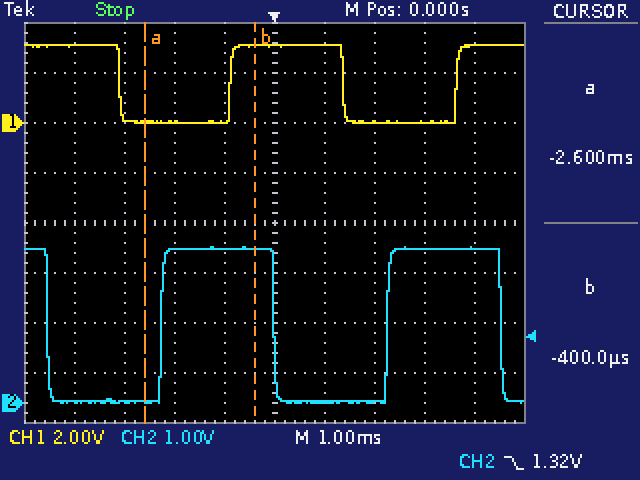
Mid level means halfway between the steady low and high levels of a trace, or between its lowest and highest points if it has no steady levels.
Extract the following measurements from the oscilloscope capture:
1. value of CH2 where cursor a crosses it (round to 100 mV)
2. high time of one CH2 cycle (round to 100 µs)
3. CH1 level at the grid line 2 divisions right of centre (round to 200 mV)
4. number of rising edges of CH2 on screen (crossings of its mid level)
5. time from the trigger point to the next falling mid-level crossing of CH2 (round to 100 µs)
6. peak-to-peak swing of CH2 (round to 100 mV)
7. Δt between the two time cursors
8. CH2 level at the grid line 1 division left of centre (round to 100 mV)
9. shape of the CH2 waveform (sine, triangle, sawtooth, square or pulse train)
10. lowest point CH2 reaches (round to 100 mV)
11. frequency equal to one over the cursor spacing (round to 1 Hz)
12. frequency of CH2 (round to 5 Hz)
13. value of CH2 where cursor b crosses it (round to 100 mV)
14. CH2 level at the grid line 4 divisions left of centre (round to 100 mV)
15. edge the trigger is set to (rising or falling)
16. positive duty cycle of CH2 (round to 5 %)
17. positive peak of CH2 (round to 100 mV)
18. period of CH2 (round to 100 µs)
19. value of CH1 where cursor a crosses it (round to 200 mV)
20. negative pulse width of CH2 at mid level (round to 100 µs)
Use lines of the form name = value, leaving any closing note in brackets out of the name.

value of CH2 where cursor a crosses it = 0.0 V
high time of one CH2 cycle = 2.3 ms
CH1 level at the grid line 2 divisions right of centre = 0.0 V
number of rising edges of CH2 on screen = 2
time from the trigger point to the next falling mid-level crossing of CH2 = 4.5 ms
peak-to-peak swing of CH2 = 3.1 V
Δt between the two time cursors = 2.2 ms
CH2 level at the grid line 1 division left of centre = 3.1 V
shape of the CH2 waveform = square
lowest point CH2 reaches = 0.0 V
frequency equal to one over the cursor spacing = 455 Hz
frequency of CH2 = 220 Hz
value of CH2 where cursor b crosses it = 3.1 V
CH2 level at the grid line 4 divisions left of centre = 0.0 V
edge the trigger is set to = falling
positive duty cycle of CH2 = 50 %
positive peak of CH2 = 3.1 V
period of CH2 = 4.5 ms
value of CH1 where cursor a crosses it = 0.0 V
negative pulse width of CH2 at mid level = 2.3 ms
